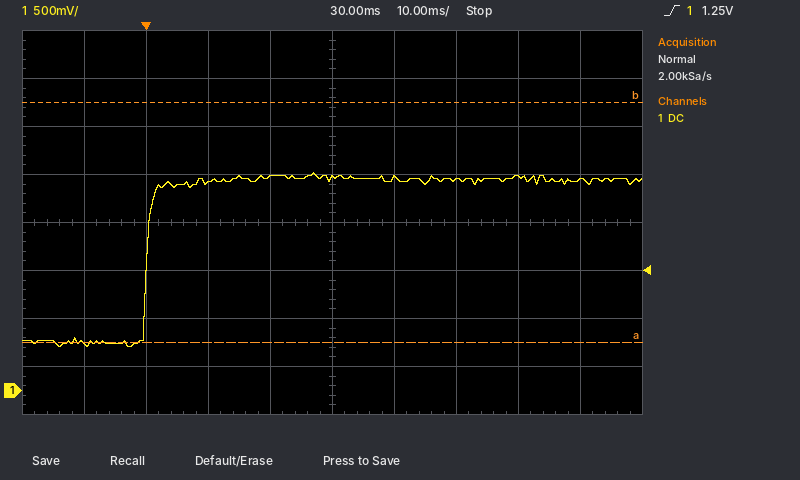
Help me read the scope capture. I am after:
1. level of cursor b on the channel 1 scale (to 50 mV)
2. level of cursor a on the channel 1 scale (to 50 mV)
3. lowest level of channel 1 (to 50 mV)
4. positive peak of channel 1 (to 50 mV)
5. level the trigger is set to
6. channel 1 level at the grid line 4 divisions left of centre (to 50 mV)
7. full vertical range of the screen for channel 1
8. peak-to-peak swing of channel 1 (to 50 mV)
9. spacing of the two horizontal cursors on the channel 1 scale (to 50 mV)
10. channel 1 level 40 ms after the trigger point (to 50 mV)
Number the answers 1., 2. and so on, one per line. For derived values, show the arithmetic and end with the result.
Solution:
1. 3.00 V
2. 500 mV
3. 450 mV
4. 2.25 V
5. 1.25 V
6. 500 mV
7. 4 V
8. 2.25 V − (450 mV) = 1.80 V
9. 2.50 V
10. 2.20 V
